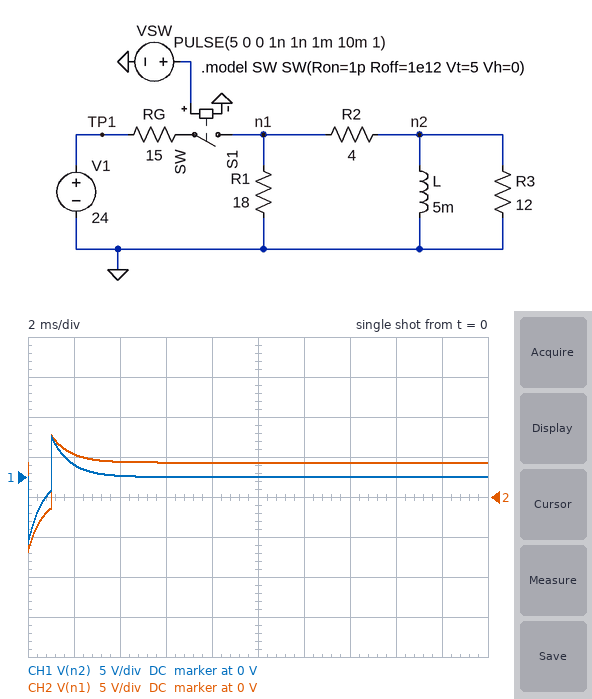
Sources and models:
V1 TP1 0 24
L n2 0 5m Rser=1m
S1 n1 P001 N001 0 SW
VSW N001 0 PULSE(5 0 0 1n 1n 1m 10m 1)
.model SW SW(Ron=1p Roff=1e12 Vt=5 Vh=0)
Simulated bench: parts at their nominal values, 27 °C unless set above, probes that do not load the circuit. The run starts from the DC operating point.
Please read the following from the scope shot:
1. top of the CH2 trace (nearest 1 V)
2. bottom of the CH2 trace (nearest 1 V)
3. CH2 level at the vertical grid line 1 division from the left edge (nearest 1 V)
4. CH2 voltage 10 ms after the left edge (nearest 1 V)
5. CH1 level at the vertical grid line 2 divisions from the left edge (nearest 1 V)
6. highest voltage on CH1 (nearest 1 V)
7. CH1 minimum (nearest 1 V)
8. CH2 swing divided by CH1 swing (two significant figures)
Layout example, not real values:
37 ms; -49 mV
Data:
8 V; -7 V; 5 V; 4 V; 0 V; 5 V; -8 V; 1.1
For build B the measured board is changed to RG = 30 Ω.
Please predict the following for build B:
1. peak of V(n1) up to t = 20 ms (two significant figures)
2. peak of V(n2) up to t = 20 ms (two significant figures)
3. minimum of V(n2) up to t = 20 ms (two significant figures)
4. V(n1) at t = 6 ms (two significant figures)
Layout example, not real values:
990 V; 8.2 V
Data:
4.7 V; 3.1 V; -4.6 V; 2.4 V
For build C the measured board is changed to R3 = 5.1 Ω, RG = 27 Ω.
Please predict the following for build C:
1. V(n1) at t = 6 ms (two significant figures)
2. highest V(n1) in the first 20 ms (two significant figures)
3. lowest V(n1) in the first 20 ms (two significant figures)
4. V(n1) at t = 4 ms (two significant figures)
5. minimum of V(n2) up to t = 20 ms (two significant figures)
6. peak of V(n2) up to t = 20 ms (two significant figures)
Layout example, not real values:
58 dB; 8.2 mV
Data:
2.6 V; 3.6 V; -2.2 V; 2.7 V; -2.7 V; 1.4 V
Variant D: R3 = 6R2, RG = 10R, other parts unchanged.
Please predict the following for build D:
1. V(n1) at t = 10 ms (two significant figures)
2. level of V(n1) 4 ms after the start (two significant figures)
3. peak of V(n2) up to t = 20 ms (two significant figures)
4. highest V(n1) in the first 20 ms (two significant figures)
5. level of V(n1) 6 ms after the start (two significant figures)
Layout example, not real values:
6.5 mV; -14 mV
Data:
5.9 V; 6.1 V; 3.6 V; 8.1 V; 6.0 V
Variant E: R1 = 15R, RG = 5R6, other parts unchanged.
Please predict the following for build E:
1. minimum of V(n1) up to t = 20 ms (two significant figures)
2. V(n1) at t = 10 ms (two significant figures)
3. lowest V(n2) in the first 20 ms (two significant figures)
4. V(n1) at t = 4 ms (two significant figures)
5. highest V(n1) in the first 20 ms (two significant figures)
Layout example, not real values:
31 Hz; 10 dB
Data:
-13 V; 8.7 V; -16 V; 8.9 V; 13 V
